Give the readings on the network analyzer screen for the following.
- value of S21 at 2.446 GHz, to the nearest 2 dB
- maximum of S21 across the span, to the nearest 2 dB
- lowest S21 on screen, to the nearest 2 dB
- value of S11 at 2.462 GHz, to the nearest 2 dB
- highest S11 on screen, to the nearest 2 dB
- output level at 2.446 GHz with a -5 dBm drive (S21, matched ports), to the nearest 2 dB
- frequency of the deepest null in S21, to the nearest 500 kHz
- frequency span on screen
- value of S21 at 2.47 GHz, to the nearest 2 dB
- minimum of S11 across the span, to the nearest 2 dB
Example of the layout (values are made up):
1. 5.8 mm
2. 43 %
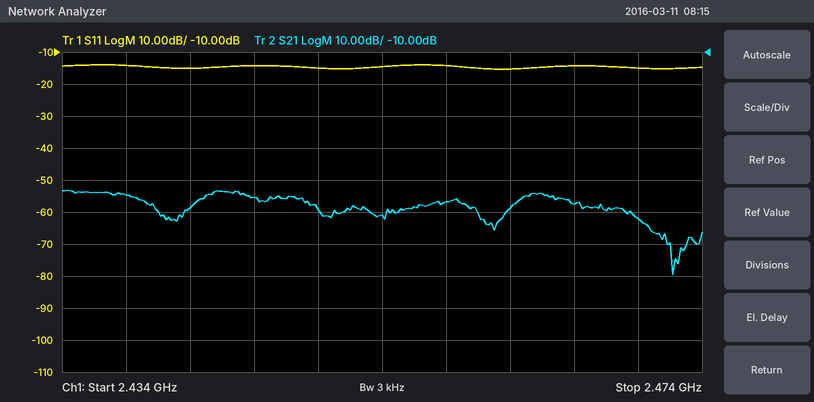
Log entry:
1. -56 dB
2. -54 dB
3. -80 dB
4. -16 dB
5. -14 dB
6. -60 dBm
7. 2.4720 GHz
8. 40 MHz
9. -62 dB
10. -16 dB
